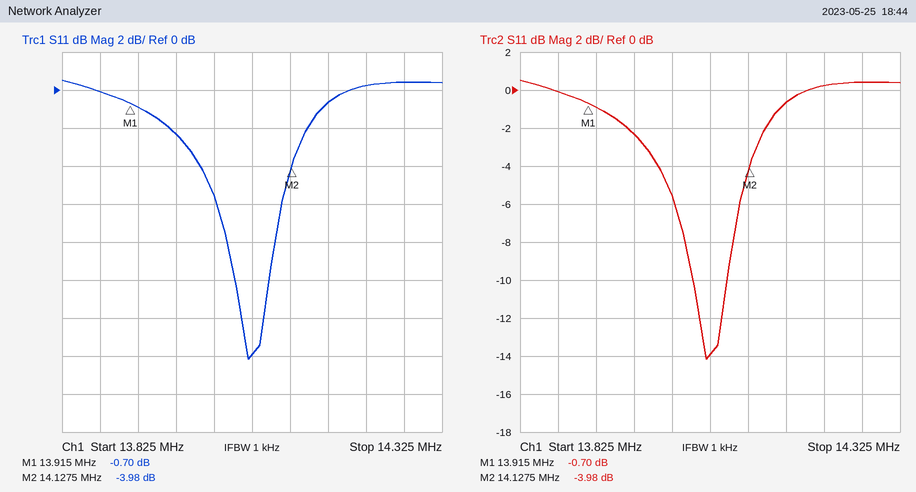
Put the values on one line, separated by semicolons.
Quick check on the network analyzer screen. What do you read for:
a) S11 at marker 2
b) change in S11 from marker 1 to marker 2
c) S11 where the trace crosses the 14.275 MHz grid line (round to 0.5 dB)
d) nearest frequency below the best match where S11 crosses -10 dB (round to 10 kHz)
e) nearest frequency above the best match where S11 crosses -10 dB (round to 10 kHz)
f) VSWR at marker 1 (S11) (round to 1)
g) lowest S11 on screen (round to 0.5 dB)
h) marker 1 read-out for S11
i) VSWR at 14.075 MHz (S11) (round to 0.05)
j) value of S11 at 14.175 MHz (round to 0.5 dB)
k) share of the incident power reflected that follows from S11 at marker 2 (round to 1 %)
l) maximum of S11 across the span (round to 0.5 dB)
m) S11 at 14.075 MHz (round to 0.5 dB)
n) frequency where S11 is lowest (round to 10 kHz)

-3.98 dB; -3.28 dB; 0.5 dB; 14.05 MHz; 14.10 MHz; 25; -14.0 dB; -0.70 dB; 1.50; -0.5 dB; 40 %; 0.5 dB; -14.0 dB; 14.07 MHz
